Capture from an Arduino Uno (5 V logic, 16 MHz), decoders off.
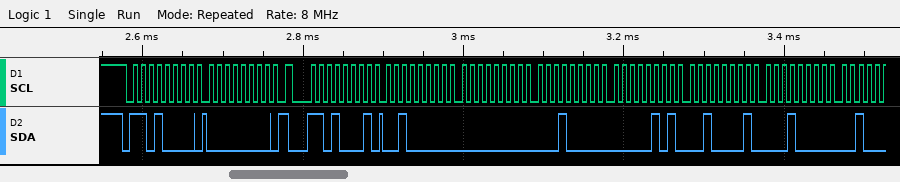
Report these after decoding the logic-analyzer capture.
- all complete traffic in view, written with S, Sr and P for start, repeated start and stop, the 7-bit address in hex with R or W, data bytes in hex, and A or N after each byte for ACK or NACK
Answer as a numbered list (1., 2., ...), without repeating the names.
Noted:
1. S 68W A 00 A Sr 68R A 20 A 00 A 10 A 05 A 21 A 10 A
